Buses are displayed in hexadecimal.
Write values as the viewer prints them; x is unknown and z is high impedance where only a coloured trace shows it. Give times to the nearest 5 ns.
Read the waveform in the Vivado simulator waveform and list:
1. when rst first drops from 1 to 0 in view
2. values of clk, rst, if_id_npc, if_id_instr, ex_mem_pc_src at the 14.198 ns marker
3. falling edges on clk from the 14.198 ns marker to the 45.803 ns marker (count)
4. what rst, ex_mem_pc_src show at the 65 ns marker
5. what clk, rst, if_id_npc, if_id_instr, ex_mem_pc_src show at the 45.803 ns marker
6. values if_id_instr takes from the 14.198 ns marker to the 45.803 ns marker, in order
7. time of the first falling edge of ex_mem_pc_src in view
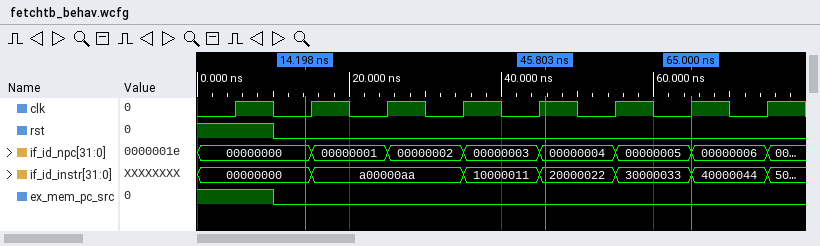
10 ns
clk=0, rst=0, if_id_npc=00000000, if_id_instr=00000000, ex_mem_pc_src=0
3
rst=0, ex_mem_pc_src=0
clk=1, rst=0, if_id_npc=00000004, if_id_instr=20000022, ex_mem_pc_src=0
00000000, a00000aa, 10000011, 20000022
10 ns
